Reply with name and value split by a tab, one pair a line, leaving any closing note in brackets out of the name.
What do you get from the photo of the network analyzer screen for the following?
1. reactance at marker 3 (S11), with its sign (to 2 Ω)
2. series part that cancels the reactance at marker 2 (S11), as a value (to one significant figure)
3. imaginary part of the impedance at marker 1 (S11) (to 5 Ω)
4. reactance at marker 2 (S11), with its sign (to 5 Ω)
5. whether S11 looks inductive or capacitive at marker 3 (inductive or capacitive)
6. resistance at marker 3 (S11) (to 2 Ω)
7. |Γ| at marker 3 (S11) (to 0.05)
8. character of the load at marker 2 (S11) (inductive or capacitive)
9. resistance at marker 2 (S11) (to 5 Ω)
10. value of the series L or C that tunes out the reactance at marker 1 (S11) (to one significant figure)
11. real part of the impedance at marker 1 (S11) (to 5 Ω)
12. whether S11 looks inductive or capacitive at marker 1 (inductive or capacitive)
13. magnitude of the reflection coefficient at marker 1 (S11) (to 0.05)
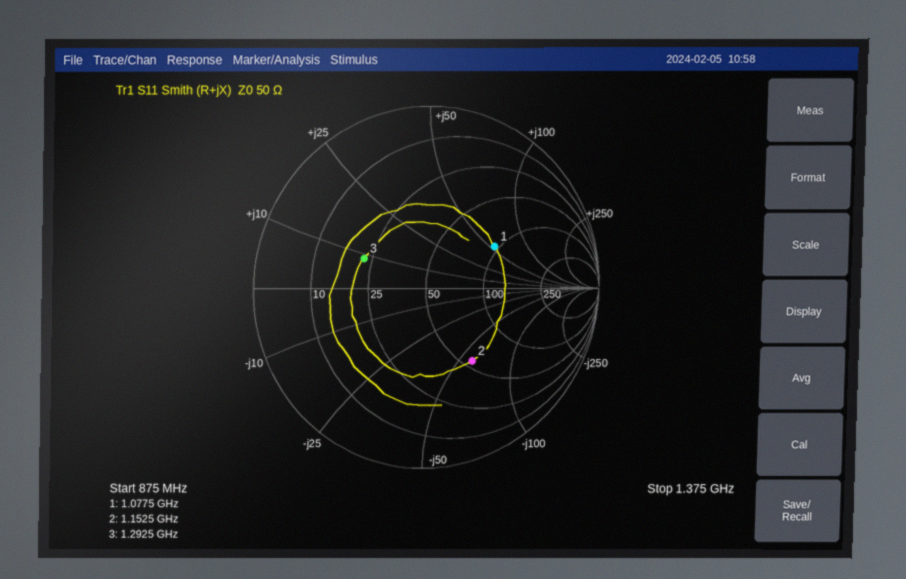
reactance at marker 3 (S11), with its sign	+8 Ω
series part that cancels the reactance at marker 2 (S11), as a value	8 nH
imaginary part of the impedance at marker 1 (S11)	+55 Ω
reactance at marker 2 (S11), with its sign	-60 Ω
whether S11 looks inductive or capacitive at marker 3	inductive
resistance at marker 3 (S11)	22 Ω
|Γ| at marker 3 (S11)	0.40
character of the load at marker 2 (S11)	capacitive
resistance at marker 2 (S11)	55 Ω
value of the series L or C that tunes out the reactance at marker 1 (S11)	3 pF
real part of the impedance at marker 1 (S11)	95 Ω
whether S11 looks inductive or capacitive at marker 1	inductive
magnitude of the reflection coefficient at marker 1 (S11)	0.45
